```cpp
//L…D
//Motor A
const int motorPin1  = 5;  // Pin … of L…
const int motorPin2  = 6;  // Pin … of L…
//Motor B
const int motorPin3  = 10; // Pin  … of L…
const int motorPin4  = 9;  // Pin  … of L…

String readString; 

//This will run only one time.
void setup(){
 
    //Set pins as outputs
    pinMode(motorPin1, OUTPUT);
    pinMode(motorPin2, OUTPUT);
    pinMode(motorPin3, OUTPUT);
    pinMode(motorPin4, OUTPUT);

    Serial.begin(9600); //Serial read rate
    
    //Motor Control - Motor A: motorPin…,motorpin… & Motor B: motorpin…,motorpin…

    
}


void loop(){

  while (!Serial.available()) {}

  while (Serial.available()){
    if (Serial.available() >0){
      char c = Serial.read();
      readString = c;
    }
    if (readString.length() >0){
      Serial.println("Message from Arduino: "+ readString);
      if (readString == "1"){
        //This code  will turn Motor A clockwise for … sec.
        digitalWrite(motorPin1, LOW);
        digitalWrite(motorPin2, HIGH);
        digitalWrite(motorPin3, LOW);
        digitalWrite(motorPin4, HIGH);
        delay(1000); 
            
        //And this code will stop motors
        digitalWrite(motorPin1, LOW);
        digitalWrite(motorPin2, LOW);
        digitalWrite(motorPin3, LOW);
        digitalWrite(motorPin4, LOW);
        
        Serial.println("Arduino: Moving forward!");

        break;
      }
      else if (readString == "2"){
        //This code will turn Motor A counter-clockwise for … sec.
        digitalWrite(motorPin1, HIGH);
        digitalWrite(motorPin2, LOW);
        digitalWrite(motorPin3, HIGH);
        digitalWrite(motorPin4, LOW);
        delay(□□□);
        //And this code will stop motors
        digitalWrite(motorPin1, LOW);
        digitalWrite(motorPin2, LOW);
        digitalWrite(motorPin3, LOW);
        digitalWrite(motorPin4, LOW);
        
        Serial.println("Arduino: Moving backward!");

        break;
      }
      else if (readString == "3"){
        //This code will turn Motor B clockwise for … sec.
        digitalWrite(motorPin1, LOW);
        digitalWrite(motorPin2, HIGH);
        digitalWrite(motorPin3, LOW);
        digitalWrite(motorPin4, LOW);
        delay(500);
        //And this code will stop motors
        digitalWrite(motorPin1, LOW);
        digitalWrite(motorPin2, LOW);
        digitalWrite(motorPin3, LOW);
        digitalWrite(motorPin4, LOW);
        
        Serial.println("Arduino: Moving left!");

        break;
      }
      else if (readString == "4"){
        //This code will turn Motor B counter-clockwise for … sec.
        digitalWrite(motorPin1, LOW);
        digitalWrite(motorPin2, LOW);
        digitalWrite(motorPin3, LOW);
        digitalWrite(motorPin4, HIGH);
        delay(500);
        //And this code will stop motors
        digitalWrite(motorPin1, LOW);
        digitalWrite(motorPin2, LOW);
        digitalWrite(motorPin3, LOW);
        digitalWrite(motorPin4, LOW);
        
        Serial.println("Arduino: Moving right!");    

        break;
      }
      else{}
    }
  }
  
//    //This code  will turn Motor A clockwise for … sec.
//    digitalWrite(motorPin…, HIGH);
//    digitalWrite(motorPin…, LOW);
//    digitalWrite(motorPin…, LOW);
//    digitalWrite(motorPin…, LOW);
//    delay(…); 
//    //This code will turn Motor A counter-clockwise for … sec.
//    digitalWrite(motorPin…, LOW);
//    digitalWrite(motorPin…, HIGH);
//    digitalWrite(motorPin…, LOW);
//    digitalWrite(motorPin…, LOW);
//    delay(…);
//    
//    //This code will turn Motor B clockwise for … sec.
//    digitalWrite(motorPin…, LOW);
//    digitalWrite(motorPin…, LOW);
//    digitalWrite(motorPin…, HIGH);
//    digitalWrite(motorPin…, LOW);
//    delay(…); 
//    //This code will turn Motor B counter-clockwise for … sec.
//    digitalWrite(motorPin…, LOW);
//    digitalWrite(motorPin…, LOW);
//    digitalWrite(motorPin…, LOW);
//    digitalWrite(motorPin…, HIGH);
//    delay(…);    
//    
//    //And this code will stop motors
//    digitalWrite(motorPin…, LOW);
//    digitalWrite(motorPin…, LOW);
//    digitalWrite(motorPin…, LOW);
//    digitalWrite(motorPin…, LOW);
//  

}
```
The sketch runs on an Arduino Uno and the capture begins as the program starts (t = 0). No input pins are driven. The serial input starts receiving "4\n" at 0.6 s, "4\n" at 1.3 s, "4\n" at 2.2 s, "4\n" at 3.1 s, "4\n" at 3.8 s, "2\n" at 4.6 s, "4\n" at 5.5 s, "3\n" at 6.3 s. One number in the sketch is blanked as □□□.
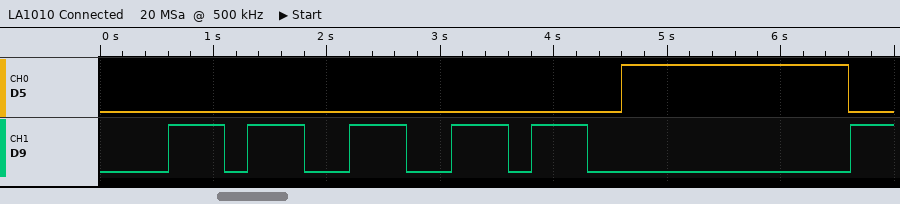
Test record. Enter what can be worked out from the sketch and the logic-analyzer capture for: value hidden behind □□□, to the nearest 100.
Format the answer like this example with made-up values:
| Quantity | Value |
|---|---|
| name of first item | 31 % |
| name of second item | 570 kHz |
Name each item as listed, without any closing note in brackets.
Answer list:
| Quantity | Value |
|---|---|
| value hidden behind □□□, to the nearest 100 | 2000 |
